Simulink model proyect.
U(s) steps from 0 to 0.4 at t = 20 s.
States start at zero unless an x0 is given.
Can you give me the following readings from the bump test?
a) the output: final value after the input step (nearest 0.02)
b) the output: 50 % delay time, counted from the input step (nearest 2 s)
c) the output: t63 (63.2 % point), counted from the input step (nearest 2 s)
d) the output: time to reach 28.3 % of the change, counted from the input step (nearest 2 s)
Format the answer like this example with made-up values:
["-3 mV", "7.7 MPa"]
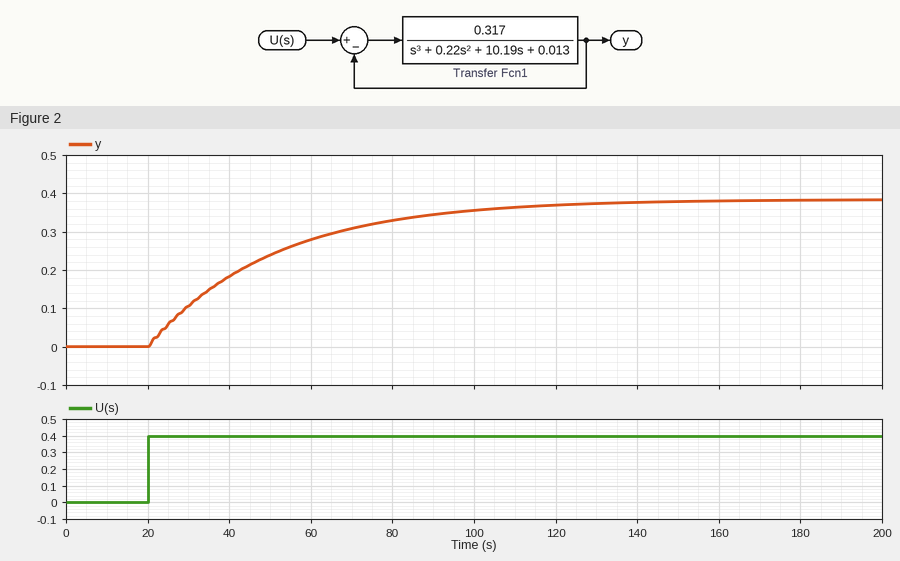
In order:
["0.38", "22 s", "30 s", "10 s"]
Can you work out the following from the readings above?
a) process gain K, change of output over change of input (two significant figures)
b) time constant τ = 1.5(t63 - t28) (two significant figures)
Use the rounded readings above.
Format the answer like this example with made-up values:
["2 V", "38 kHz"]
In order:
["0.95", "30 s"]
